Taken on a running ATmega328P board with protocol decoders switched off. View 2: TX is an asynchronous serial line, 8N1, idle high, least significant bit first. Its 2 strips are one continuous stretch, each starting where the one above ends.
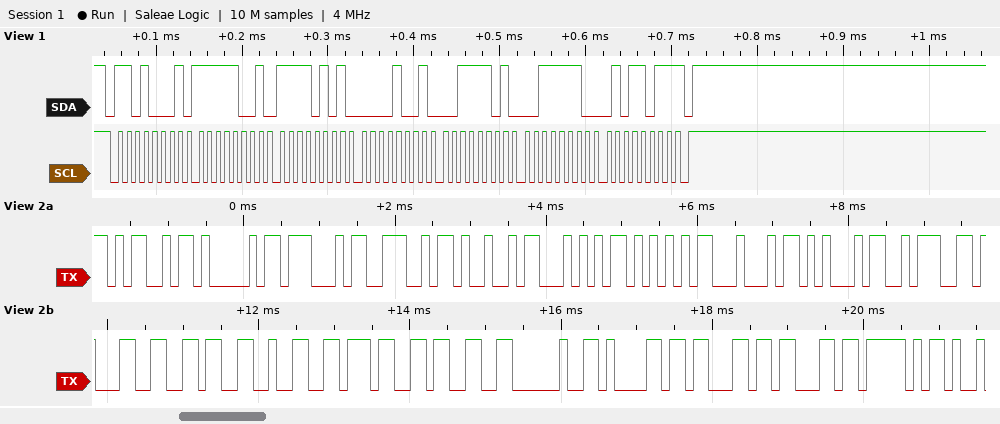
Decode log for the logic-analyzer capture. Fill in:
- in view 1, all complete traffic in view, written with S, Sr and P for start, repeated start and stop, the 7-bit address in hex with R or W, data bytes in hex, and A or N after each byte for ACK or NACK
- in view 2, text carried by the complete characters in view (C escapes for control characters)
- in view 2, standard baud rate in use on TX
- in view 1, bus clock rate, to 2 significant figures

S 68R A F9 A F5 A 09 A 3D A 3E A 5B N P
"MAGNITUDE:16273 acc_"
9600 baud
100 kHz
